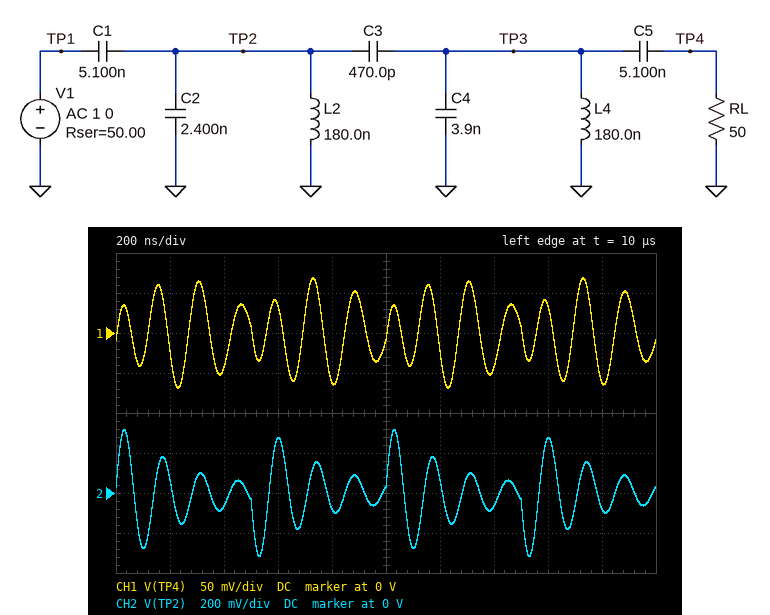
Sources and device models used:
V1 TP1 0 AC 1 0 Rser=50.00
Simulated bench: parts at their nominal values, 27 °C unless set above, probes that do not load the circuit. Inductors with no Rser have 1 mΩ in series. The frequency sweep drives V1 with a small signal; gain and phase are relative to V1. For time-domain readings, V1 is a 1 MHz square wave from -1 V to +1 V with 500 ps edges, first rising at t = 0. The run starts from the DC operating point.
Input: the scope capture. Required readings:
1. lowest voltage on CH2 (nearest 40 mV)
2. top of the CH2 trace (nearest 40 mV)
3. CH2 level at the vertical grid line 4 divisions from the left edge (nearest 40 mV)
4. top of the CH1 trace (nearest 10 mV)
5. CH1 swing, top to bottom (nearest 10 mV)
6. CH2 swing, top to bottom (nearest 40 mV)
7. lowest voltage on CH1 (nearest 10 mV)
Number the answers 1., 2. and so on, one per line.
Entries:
1. -320 mV
2. 320 mV
3. -80 mV
4. 70 mV
5. 140 mV
6. 640 mV
7. -70 mV
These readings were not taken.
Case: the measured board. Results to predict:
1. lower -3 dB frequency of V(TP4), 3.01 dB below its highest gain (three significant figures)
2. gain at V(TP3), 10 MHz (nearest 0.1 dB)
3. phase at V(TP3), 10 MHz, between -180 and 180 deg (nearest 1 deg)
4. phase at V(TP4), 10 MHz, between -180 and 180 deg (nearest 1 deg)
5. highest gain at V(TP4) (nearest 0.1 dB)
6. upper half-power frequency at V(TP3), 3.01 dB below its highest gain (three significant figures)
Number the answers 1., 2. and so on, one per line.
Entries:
1. 5.36 MHz
2. -29.3 dB
3. -67 deg
4. -64 deg
5. -11.5 dB
6. 7.51 MHz
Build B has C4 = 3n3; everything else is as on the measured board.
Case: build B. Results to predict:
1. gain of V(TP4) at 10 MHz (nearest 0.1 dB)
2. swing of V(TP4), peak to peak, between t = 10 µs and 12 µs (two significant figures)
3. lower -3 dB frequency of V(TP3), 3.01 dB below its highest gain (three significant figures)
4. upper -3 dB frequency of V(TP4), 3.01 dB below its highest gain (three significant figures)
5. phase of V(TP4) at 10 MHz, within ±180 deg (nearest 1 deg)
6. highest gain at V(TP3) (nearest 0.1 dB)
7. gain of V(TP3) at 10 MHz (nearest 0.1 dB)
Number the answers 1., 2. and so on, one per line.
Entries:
1. -27.3 dB
2. 160 mV
3. 5.72 MHz
4. 7.56 MHz
5. -62 deg
6. -8.8 dB
7. -27.2 dB
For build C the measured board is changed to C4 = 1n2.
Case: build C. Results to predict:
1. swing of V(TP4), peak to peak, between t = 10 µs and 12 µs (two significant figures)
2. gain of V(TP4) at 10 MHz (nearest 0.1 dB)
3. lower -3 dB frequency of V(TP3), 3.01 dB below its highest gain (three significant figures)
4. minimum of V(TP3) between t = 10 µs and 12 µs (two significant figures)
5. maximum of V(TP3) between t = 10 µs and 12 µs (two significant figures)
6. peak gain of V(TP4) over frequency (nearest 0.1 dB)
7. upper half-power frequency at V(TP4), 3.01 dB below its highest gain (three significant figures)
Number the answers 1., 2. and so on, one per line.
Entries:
1. 250 mV
2. -11.6 dB
3. 6.47 MHz
4. -120 mV
5. 120 mV
6. -10.2 dB
7. 10.4 MHz
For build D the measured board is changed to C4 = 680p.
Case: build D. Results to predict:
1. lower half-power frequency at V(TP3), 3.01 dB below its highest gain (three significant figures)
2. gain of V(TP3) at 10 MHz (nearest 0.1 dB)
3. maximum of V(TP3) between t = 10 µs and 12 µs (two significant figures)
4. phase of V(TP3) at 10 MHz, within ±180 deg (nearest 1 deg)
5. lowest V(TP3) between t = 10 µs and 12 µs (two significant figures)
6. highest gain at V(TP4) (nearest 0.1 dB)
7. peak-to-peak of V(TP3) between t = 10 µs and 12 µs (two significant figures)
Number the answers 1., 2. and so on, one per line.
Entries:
1. 6.48 MHz
2. -14.4 dB
3. 110 mV
4. 63 deg
5. -110 mV
6. -12.4 dB
7. 230 mV
